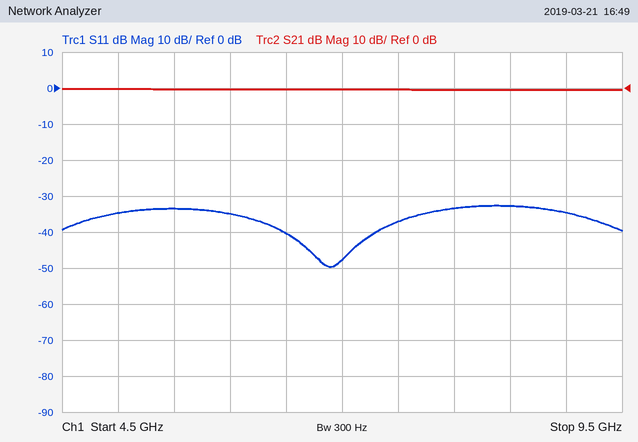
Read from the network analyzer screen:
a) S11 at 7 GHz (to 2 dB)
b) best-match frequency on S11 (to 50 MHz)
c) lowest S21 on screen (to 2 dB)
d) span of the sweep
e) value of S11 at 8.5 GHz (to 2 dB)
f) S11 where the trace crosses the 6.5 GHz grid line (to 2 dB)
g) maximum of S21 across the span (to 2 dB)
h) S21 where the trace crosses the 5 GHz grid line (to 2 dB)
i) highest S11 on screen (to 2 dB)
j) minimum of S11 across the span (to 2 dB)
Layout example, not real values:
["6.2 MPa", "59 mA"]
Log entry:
["-48 dB", "6.90 GHz", "0 dB", "5 GHz", "-32 dB", "-40 dB", "0 dB", "0 dB", "-32 dB", "-50 dB"]
